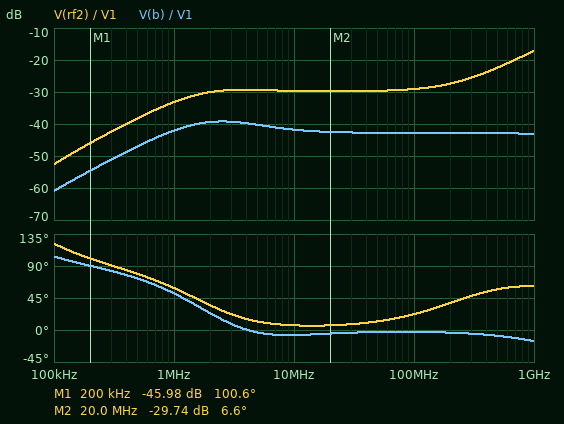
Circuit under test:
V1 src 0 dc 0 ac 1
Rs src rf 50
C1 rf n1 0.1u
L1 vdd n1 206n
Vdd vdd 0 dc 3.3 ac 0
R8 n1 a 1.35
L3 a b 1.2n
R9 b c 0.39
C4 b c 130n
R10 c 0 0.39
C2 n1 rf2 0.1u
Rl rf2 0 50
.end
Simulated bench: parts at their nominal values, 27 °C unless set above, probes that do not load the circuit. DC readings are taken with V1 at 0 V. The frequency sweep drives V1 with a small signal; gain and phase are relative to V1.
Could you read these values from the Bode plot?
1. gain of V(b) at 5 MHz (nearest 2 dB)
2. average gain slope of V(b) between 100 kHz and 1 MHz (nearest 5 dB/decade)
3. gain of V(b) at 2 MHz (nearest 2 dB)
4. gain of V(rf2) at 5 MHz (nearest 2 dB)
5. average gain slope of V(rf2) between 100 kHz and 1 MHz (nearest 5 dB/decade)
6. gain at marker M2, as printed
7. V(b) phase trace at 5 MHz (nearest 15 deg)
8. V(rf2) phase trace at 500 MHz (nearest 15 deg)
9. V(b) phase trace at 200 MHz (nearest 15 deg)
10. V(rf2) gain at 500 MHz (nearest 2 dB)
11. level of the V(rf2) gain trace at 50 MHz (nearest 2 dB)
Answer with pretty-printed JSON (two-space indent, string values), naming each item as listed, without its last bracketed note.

{
  "gain of V(b) at 5 MHz": "-40 dB",
  "average gain slope of V(b) between 100 kHz and 1 MHz": "20 dB/decade",
  "gain of V(b) at 2 MHz": "-40 dB",
  "gain of V(rf2) at 5 MHz": "-30 dB",
  "average gain slope of V(rf2) between 100 kHz and 1 MHz": "20 dB/decade",
  "gain at marker M2, as printed": "-29.74 dB",
  "V(b) phase trace at 5 MHz": "0 deg",
  "V(rf2) phase trace at 500 MHz": "60 deg",
  "V(b) phase trace at 200 MHz": "0 deg",
  "V(rf2) gain at 500 MHz": "-22 dB",
  "level of the V(rf2) gain trace at 50 MHz": "-30 dB"
}
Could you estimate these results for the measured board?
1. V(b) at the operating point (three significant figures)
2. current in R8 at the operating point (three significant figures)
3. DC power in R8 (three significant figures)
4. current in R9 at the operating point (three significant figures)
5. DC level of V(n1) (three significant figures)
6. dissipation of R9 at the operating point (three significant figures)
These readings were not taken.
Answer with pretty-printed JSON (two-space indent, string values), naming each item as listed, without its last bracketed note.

{
  "V(b) at the operating point": "1.21 V",
  "current in R8 at the operating point": "1.55 A",
  "DC power in R8": "3.24 W",
  "current in R9 at the operating point": "1.55 A",
  "DC level of V(n1)": "3.30 V",
  "dissipation of R9 at the operating point": "936 mW"
}
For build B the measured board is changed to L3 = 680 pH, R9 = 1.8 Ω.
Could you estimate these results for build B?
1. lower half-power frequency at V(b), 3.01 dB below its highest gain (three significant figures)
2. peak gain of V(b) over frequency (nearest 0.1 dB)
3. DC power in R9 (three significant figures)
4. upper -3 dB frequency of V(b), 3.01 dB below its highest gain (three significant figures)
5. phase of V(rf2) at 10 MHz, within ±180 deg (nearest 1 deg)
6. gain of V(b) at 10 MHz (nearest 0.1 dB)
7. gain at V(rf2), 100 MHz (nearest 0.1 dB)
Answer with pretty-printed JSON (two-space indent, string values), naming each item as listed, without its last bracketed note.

{
  "lower half-power frequency at V(b), 3.01 dB below its highest gain": "694 kHz",
  "peak gain of V(b) over frequency": "-36.5 dB",
  "DC power in R9": "1.56 W",
  "upper -3 dB frequency of V(b), 3.01 dB below its highest gain": "3.45 MHz",
  "phase of V(rf2) at 10 MHz, within ±180 deg": "5 deg",
  "gain of V(b) at 10 MHz": "-42.2 dB",
  "gain at V(rf2), 100 MHz": "-29.5 dB"
}
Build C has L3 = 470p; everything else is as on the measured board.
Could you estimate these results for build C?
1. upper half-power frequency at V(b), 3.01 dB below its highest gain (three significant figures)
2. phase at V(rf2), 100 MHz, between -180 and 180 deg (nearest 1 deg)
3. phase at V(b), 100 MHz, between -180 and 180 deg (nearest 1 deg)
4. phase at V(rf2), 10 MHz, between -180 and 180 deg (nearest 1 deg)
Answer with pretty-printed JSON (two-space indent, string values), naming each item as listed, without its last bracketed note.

{
  "upper half-power frequency at V(b), 3.01 dB below its highest gain": "14.1 MHz",
  "phase at V(rf2), 100 MHz, between -180 and 180 deg": "9 deg",
  "phase at V(b), 100 MHz, between -180 and 180 deg": "-2 deg",
  "phase at V(rf2), 10 MHz, between -180 and 180 deg": "5 deg"
}
